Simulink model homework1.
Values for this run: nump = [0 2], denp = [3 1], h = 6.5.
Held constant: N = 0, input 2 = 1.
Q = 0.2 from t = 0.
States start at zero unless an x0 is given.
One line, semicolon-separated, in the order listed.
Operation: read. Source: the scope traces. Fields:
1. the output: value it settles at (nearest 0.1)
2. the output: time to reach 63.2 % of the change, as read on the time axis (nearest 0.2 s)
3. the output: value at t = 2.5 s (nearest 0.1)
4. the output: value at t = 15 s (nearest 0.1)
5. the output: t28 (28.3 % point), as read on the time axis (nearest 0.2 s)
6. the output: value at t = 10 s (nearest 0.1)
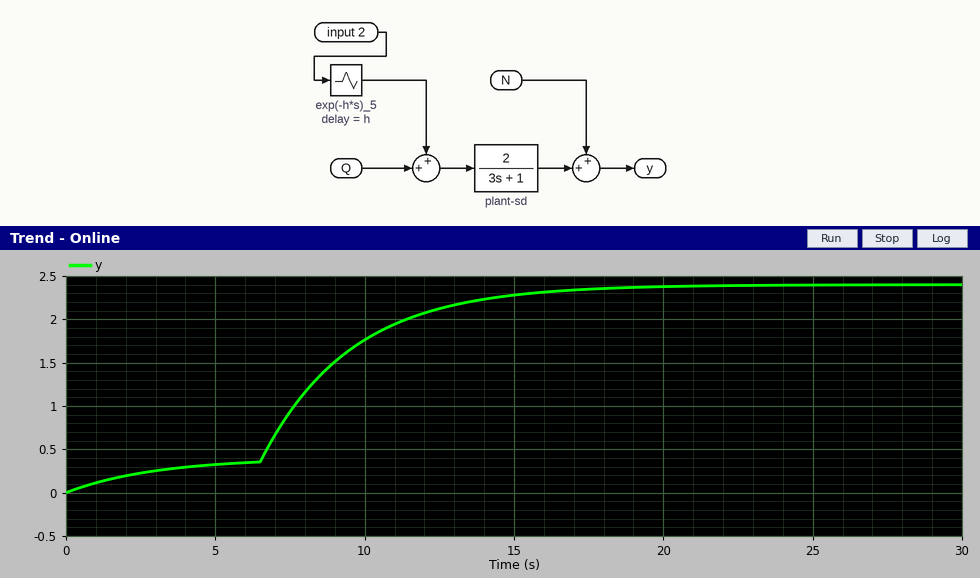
2.4; 9.0 s; 0.2; 2.3; 7.0 s; 1.8
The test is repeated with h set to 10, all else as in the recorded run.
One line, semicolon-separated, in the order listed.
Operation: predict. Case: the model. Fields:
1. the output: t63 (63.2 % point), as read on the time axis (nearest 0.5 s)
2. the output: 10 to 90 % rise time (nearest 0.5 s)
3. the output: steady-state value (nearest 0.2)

12.5 s; 13.5 s; 2.4
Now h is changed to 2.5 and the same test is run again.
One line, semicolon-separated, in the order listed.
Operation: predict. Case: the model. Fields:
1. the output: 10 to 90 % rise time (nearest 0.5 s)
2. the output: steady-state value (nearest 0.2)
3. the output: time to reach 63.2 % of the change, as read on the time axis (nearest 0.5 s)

6.5 s; 2.4; 5.0 s
